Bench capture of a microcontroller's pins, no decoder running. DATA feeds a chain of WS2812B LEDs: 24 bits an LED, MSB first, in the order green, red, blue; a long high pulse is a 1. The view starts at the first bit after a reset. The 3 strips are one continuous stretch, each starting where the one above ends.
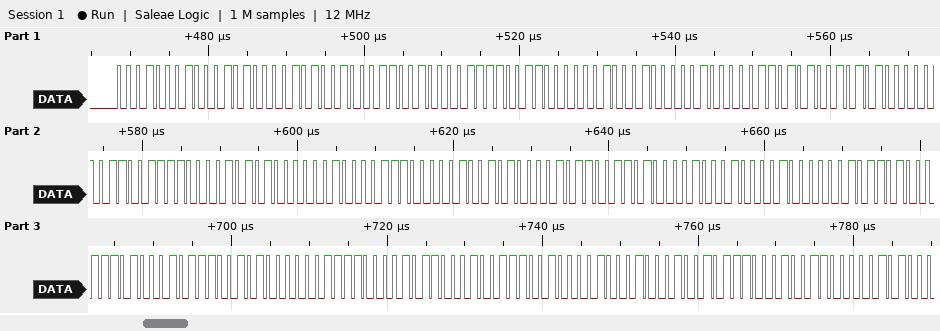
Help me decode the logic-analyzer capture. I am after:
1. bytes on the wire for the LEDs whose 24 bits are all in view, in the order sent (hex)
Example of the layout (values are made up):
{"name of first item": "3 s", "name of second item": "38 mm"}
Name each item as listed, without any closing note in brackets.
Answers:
{"bytes on the wire for the LEDs whose 24 bits are all in view, in the order sent": "11 14 29 19 0F 30 22 08 35 2A 03 3C 2A 04 38 25 0B 34 22 10 2D 1D 17 28 1E 16 27 21 11 2E"}
